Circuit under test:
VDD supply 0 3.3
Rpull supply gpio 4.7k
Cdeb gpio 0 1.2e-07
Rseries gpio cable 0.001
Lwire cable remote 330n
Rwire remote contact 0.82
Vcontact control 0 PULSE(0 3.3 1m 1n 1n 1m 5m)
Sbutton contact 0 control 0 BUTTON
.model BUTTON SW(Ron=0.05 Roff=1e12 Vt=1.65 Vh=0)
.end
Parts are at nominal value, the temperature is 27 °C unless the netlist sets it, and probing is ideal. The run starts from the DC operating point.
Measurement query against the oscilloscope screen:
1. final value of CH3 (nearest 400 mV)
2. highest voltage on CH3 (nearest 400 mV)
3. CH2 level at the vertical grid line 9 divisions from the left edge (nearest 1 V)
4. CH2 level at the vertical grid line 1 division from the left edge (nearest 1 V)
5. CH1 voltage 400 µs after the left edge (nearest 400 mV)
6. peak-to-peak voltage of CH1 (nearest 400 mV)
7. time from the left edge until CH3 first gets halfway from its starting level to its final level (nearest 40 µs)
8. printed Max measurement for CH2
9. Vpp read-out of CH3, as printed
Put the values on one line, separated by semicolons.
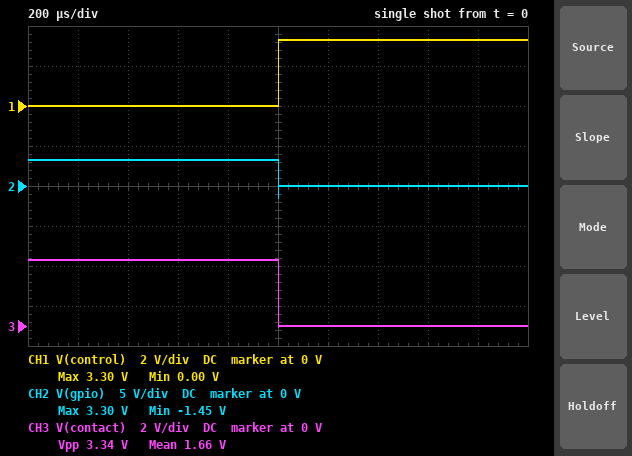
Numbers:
0 V; 3.2 V; 0 V; 3 V; 0 V; 3.2 V; 1.00 ms; 3.30 V; 3.34 V
